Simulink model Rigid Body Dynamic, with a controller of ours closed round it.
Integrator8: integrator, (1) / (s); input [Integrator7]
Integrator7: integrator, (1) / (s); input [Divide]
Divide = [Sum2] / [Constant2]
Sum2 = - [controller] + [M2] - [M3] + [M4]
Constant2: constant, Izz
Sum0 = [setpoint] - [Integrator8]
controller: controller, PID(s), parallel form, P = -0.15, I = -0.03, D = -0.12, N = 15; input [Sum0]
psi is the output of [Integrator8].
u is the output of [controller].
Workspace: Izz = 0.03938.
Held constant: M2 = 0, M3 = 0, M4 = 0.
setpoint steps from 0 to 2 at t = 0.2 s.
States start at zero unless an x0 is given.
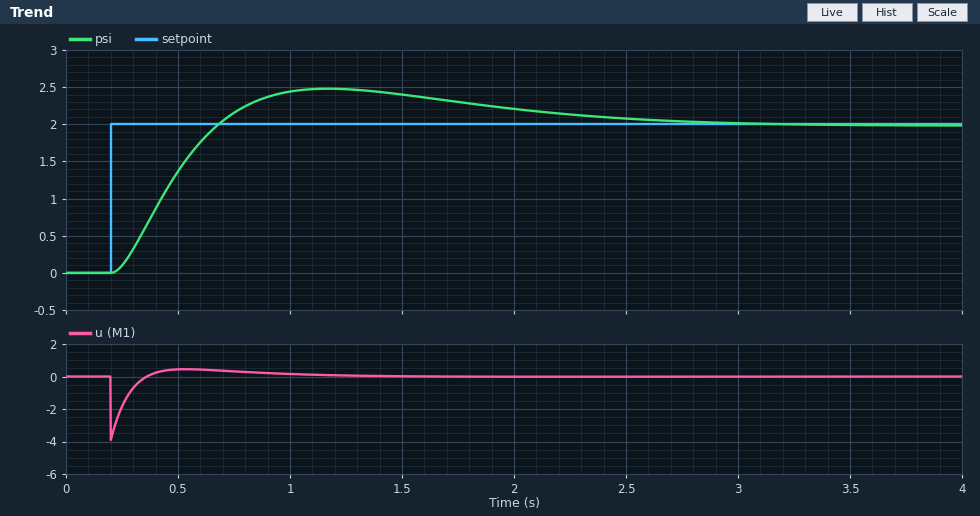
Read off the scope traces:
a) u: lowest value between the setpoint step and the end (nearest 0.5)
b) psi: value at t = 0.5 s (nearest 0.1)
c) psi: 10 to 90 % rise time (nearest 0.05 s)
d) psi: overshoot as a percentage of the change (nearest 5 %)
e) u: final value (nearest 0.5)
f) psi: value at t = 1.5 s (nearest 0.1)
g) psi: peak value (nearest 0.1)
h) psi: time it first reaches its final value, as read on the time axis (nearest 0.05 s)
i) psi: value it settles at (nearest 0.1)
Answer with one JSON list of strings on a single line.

["-4.0", "1.4", "0.35 s", "25 %", "0.0", "2.4", "2.5", "0.70 s", "2.0"]
